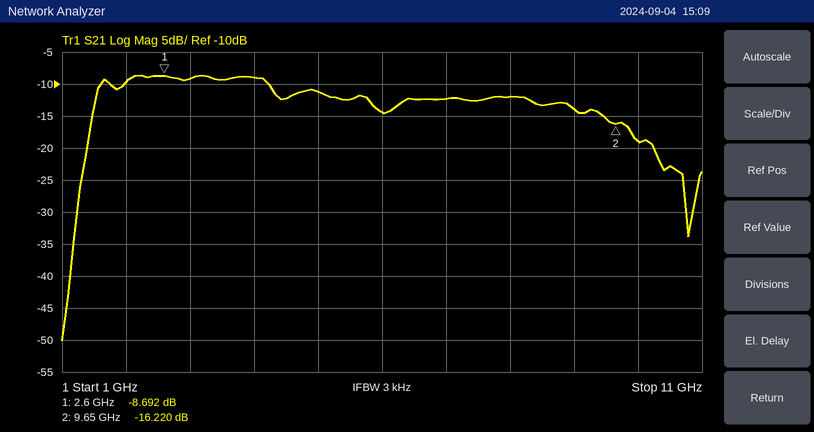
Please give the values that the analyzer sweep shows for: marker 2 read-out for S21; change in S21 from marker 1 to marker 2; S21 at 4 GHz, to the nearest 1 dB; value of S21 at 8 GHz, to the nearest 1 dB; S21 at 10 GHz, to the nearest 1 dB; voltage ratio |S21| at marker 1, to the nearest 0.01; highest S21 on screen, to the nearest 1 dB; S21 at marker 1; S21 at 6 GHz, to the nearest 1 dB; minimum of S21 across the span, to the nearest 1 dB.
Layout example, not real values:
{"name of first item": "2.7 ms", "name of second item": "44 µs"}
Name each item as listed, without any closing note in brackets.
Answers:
{"marker 2 read-out for S21": "-16.220 dB", "change in S21 from marker 1 to marker 2": "-7.528 dB", "S21 at 4 GHz, to the nearest 1 dB": "-9 dB", "value of S21 at 8 GHz, to the nearest 1 dB": "-12 dB", "S21 at 10 GHz, to the nearest 1 dB": "-19 dB", "voltage ratio |S21| at marker 1, to the nearest 0.01": "0.37", "highest S21 on screen, to the nearest 1 dB": "-9 dB", "S21 at marker 1": "-8.692 dB", "S21 at 6 GHz, to the nearest 1 dB": "-14 dB", "minimum of S21 across the span, to the nearest 1 dB": "-50 dB"}
